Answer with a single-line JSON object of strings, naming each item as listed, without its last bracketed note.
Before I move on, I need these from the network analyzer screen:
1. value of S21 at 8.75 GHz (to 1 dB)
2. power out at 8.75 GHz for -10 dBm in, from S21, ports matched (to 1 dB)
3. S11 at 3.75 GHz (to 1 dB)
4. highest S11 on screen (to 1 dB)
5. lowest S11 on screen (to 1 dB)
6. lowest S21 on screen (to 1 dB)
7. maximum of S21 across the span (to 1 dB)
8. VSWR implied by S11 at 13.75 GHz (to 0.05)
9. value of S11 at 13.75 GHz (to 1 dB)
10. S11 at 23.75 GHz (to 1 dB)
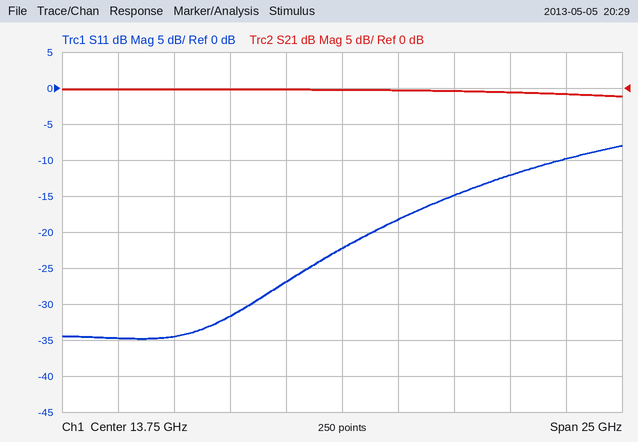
{"value of S21 at 8.75 GHz": "0 dB", "power out at 8.75 GHz for -10 dBm in, from S21, ports matched": "-10 dBm", "S11 at 3.75 GHz": "-35 dB", "highest S11 on screen": "-8 dB", "lowest S11 on screen": "-35 dB", "lowest S21 on screen": "-1 dB", "maximum of S21 across the span": "0 dB", "VSWR implied by S11 at 13.75 GHz": "1.15", "value of S11 at 13.75 GHz": "-22 dB", "S11 at 23.75 GHz": "-10 dB"}
